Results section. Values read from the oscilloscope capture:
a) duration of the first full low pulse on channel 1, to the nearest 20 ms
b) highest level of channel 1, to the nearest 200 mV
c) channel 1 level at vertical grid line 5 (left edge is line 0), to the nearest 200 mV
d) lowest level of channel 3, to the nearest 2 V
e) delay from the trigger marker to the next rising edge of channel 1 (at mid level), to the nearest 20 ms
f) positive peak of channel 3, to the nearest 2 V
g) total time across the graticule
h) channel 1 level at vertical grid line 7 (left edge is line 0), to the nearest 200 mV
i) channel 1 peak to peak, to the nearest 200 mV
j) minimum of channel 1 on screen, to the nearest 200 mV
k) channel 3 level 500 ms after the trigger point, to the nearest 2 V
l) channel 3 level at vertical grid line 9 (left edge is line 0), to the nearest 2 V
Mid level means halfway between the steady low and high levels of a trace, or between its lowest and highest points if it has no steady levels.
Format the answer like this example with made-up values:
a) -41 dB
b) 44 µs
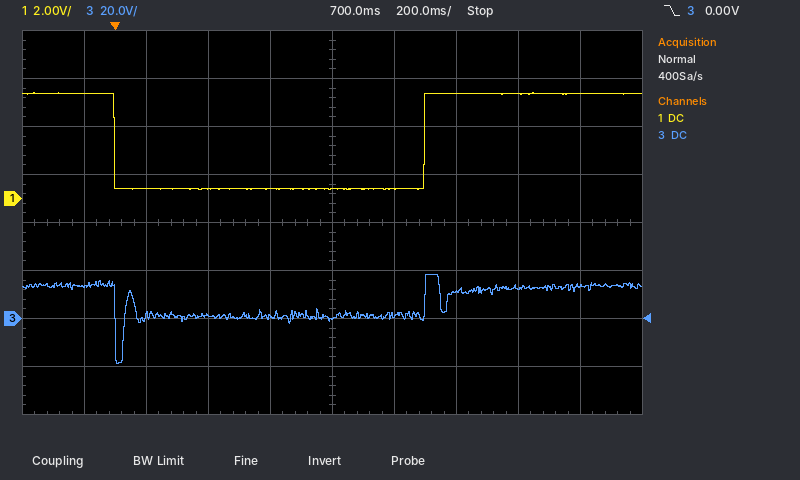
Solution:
a) 1.00 s
b) 4.4 V
c) 400 mV
d) -18 V
e) 1.00 s
f) 18 V
g) 2 s
h) 4.4 V
i) 4.0 V
j) 400 mV
k) 0 V
l) 14 V
